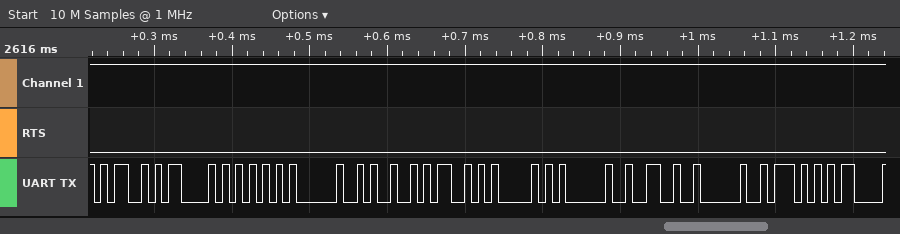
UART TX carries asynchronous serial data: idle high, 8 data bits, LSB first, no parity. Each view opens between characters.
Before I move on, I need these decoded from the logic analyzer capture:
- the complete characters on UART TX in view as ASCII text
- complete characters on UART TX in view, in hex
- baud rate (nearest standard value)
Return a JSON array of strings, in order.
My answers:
["\"MCU ISP & W\"", "4D, 43, 55, 20, 49, 53, 50, 20, 26, 20, 57", "115200 baud"]
